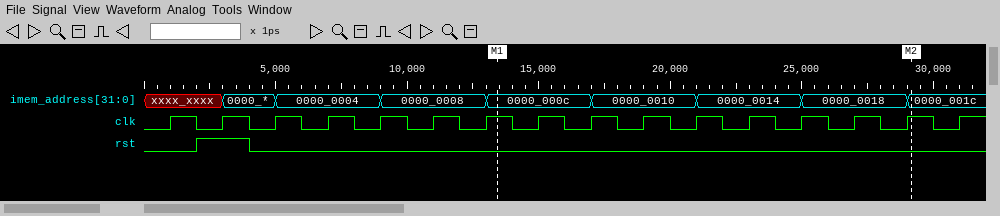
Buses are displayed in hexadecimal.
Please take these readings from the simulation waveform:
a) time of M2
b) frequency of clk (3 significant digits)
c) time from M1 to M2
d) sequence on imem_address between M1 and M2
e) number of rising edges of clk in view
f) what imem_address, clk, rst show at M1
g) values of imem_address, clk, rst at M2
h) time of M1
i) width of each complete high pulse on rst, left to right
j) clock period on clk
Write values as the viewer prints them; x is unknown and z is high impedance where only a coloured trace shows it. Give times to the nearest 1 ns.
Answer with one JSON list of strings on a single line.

["29 ns", "500 MHz", "16 ns", "0000_000c, 0000_0010, 0000_0014, 0000_0018, 0000_001c", "16", "imem_address=0000_000c, clk=1, rst=0", "imem_address=0000_001c, clk=1, rst=0", "13 ns", "2 ns", "2 ns"]
